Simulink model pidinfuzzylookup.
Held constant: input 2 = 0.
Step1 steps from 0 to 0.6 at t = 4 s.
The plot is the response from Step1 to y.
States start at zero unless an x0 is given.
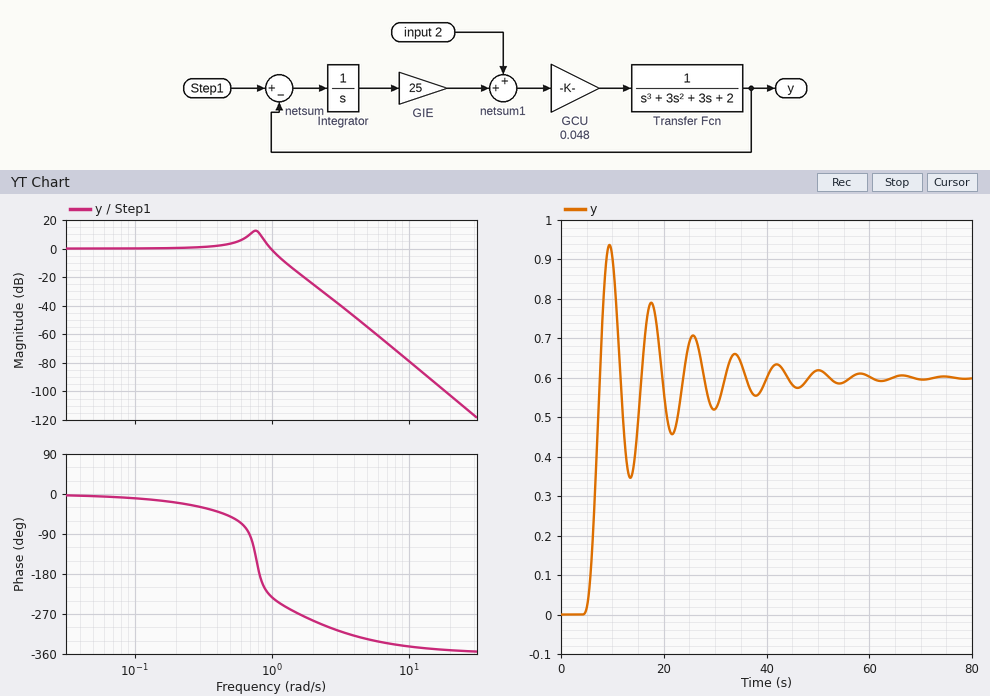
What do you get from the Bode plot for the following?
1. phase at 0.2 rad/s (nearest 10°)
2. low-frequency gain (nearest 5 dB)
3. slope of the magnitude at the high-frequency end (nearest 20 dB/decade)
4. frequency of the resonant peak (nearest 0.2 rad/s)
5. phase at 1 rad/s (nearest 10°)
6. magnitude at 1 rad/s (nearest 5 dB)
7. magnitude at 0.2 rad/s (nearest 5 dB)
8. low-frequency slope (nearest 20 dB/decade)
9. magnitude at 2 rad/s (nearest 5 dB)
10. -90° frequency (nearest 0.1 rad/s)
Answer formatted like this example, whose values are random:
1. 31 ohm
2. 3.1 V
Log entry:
1. -20°
2. 0 dB
3. -80 dB/decade
4. 0.8 rad/s
5. -230°
6. 0 dB
7. 0 dB
8. 0 dB/decade
9. -25 dB
10. 0.7 rad/s
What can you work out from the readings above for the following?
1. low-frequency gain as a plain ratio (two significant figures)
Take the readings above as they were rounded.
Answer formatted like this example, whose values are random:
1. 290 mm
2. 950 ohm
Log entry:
1. 1.0
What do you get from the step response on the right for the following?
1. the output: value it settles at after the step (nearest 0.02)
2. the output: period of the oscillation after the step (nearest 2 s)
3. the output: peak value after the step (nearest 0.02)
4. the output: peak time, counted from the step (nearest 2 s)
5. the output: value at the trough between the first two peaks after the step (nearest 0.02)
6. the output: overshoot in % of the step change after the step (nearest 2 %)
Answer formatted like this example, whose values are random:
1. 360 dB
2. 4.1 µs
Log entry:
1. 0.60
2. 8 s
3. 0.94
4. 6 s
5. 0.34
6. 56 %
